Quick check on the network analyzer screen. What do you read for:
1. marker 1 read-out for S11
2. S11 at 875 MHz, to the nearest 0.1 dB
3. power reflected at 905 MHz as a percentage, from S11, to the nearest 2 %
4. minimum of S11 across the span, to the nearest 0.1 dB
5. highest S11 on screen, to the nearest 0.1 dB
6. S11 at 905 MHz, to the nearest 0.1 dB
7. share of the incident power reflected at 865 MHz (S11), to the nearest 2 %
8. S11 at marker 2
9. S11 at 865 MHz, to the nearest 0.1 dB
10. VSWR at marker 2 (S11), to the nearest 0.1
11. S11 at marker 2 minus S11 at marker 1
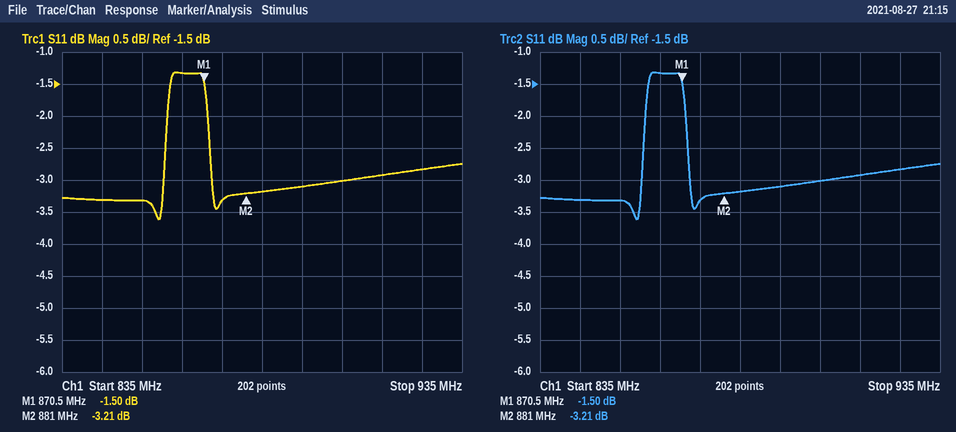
-1.50 dB
-3.3 dB
50 %
-3.6 dB
-1.3 dB
-3.0 dB
74 %
-3.21 dB
-1.3 dB
5.5
-1.71 dB
